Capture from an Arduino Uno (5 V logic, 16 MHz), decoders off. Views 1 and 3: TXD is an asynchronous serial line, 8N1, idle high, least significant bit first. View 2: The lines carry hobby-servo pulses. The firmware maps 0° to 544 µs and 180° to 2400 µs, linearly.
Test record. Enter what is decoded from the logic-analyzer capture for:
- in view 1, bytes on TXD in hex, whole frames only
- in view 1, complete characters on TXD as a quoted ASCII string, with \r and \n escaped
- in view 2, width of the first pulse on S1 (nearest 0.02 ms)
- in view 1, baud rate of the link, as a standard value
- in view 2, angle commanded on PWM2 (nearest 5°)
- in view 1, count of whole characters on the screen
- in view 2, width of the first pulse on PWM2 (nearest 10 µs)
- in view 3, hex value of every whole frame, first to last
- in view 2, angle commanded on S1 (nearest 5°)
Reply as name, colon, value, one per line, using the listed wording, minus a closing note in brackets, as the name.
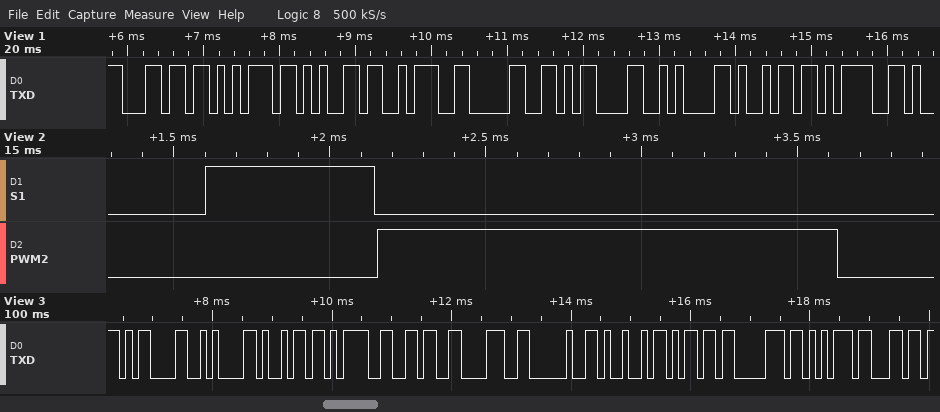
in view 1, bytes on TXD in hex, whole frames only: 6C 75 65 3A 30 0D 0A 69 3D
in view 1, complete characters on TXD as a quoted ASCII string, with \r and \n escaped: "lue:0\r\ni="
in view 2, width of the first pulse on S1: 0.54 ms
in view 1, baud rate of the link, as a standard value: 9600 baud
in view 2, angle commanded on PWM2: 90°
in view 1, count of whole characters on the screen: 9
in view 2, width of the first pulse on PWM2: 1470 µs
in view 3, hex value of every whole frame, first to last: 0D 0A 69 3D 36 38 20 49 6D 70 75 6C
in view 2, angle commanded on S1: 0°
